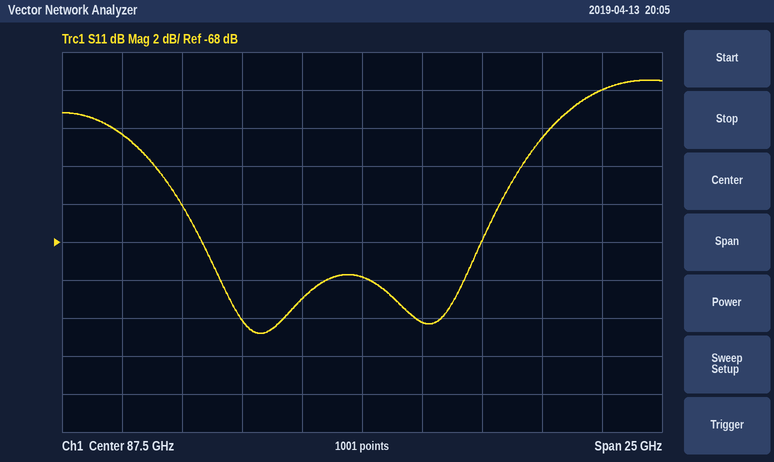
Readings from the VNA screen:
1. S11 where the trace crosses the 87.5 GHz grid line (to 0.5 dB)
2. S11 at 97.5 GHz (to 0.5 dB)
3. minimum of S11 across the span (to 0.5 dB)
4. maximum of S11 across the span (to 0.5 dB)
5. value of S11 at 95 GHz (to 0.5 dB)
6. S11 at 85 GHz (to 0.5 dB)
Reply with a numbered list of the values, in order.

1. -70.0 dB
2. -60.0 dB
3. -73.0 dB
4. -59.5 dB
5. -62.5 dB
6. -71.0 dB
